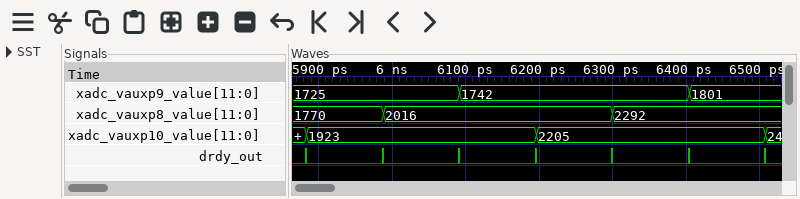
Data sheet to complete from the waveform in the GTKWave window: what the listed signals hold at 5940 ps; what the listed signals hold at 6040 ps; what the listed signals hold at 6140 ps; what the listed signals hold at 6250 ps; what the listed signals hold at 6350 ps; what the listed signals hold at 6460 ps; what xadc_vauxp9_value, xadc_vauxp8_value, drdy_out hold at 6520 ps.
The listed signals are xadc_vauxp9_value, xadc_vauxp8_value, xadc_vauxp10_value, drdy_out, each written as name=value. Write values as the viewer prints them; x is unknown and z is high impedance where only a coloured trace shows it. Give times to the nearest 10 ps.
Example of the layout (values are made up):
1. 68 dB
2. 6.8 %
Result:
1. xadc_vauxp9_value=1725, xadc_vauxp8_value=1770, xadc_vauxp10_value=1923, drdy_out=0
2. xadc_vauxp9_value=1725, xadc_vauxp8_value=2016, xadc_vauxp10_value=1923, drdy_out=0
3. xadc_vauxp9_value=1742, xadc_vauxp8_value=2016, xadc_vauxp10_value=1923, drdy_out=0
4. xadc_vauxp9_value=1742, xadc_vauxp8_value=2016, xadc_vauxp10_value=2205, drdy_out=0
5. xadc_vauxp9_value=1742, xadc_vauxp8_value=2292, xadc_vauxp10_value=2205, drdy_out=0
6. xadc_vauxp9_value=1801, xadc_vauxp8_value=2292, xadc_vauxp10_value=2205, drdy_out=0
7. xadc_vauxp9_value=1801, xadc_vauxp8_value=2292, drdy_out=0
